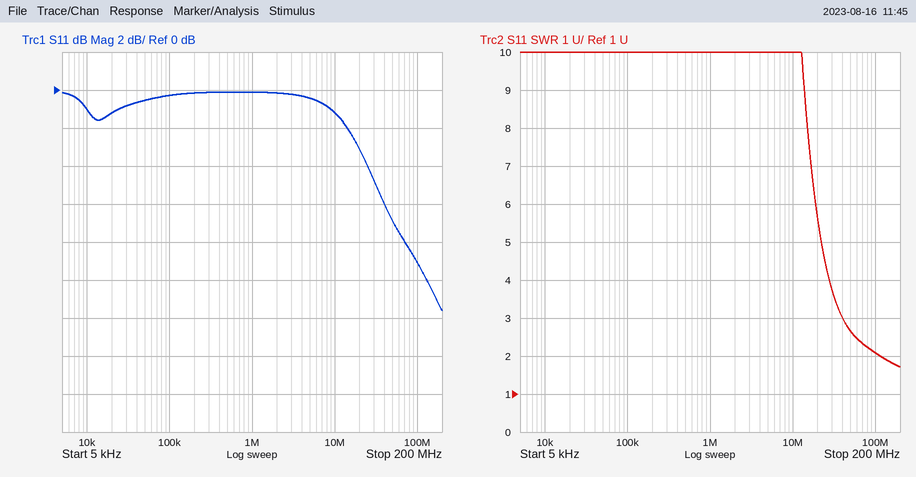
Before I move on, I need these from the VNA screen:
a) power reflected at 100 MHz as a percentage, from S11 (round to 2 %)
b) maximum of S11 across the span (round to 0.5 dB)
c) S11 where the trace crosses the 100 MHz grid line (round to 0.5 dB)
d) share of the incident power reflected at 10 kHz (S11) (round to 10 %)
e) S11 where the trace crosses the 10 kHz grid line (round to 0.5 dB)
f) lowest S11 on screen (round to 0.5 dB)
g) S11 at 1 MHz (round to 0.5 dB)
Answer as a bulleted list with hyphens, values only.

- 12 %
- 0.0 dB
- -9.0 dB
- 80 %
- -1.0 dB
- -11.5 dB
- 0.0 dB
